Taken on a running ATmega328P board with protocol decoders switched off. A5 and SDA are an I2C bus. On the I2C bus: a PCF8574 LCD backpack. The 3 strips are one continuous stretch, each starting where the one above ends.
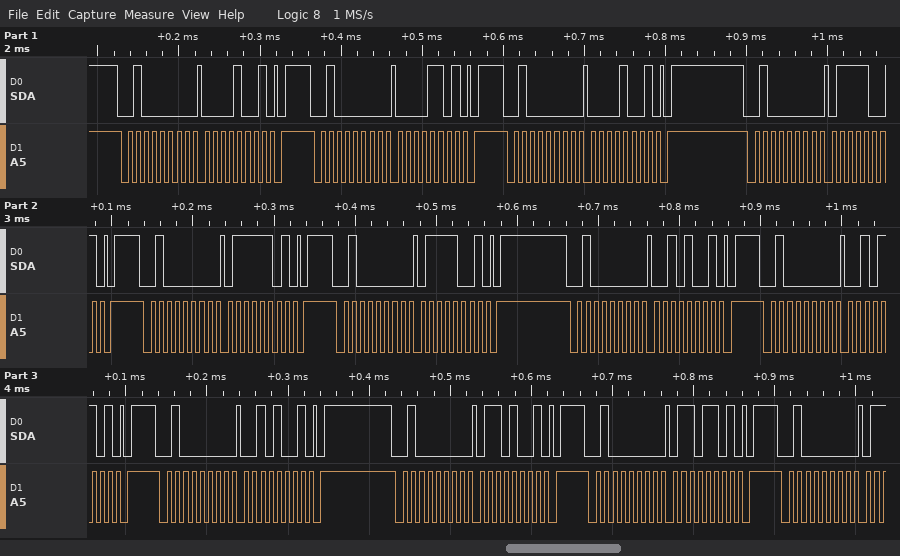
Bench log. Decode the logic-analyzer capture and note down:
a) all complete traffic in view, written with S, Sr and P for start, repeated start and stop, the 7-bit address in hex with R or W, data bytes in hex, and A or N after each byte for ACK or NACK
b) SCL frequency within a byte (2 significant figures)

S 20W A 09 A P S 20W A 0D A P S 20W A 09 A P S 20W A 79 A P S 20W A 7D A P S 20W A 79 A P S 20W A 29 A P S 20W A 2D A P S 20W A 29 A P S 20W A 69 A P S 20W A 6D A P S 20W A
100 kHz
